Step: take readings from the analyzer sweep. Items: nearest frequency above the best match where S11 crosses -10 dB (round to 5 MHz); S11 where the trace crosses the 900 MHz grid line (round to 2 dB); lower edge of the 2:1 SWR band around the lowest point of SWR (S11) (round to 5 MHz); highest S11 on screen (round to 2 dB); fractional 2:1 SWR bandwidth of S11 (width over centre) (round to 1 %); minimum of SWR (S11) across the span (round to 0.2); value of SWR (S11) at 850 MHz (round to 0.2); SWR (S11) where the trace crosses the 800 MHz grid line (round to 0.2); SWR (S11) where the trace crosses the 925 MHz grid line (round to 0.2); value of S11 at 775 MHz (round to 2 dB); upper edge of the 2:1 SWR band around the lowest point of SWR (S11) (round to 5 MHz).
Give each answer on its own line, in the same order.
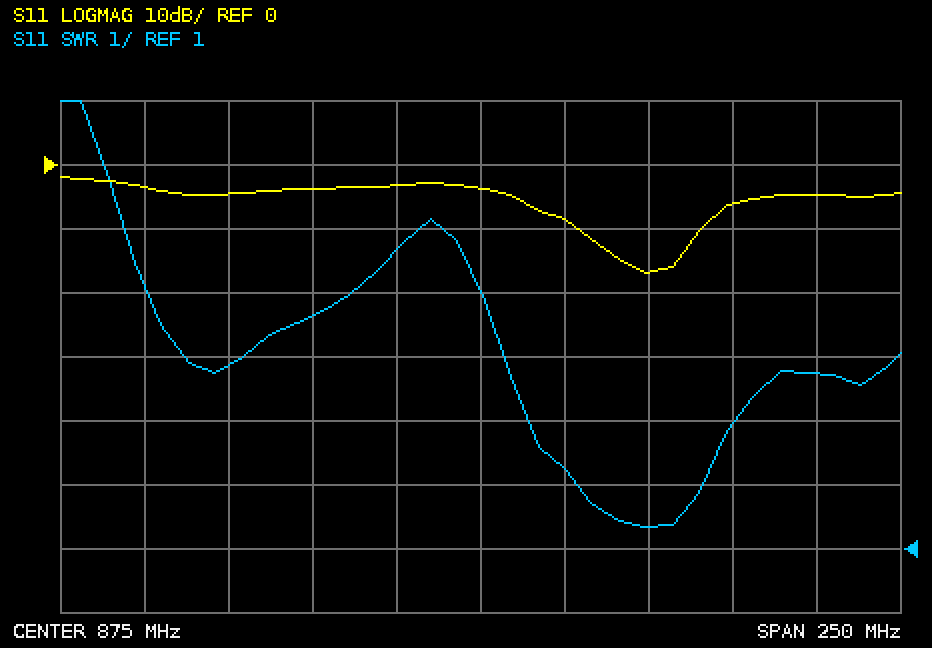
940 MHz
-8 dB
905 MHz
-2 dB
4 %
1.4
5.6
3.8
1.4
-4 dB
940 MHz
